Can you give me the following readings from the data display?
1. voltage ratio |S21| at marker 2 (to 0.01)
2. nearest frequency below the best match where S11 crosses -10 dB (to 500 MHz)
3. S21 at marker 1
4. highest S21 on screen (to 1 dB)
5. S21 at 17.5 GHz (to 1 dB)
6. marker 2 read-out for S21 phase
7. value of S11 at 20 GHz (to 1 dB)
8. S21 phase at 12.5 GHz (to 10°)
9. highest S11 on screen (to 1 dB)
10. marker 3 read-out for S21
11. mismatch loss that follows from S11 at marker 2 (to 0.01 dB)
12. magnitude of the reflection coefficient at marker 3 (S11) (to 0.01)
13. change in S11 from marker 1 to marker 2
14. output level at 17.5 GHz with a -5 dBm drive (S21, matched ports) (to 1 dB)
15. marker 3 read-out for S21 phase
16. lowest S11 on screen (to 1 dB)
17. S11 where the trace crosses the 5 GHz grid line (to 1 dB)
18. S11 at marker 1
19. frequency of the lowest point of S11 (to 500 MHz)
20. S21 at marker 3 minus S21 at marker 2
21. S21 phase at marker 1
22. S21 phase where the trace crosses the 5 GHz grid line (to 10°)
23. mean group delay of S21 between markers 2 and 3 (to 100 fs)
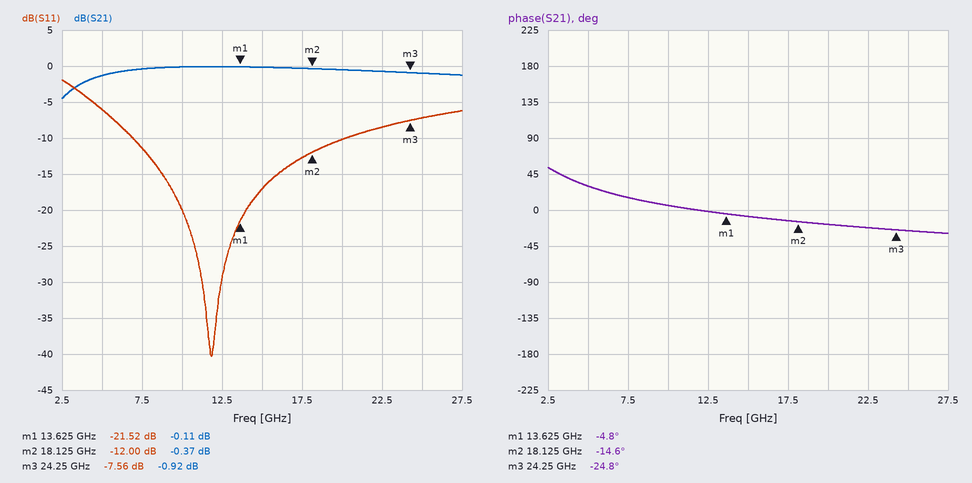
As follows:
0.96
7.0 GHz
-0.11 dB
0 dB
0 dB
-14.6°
-10 dB
0°
-2 dB
-0.92 dB
0.28 dB
0.42
9.52 dB
-5 dBm
-24.8°
-40 dB
-6 dB
-21.52 dB
12.0 GHz
-0.55 dB
-4.8°
30°
4.6 ps
